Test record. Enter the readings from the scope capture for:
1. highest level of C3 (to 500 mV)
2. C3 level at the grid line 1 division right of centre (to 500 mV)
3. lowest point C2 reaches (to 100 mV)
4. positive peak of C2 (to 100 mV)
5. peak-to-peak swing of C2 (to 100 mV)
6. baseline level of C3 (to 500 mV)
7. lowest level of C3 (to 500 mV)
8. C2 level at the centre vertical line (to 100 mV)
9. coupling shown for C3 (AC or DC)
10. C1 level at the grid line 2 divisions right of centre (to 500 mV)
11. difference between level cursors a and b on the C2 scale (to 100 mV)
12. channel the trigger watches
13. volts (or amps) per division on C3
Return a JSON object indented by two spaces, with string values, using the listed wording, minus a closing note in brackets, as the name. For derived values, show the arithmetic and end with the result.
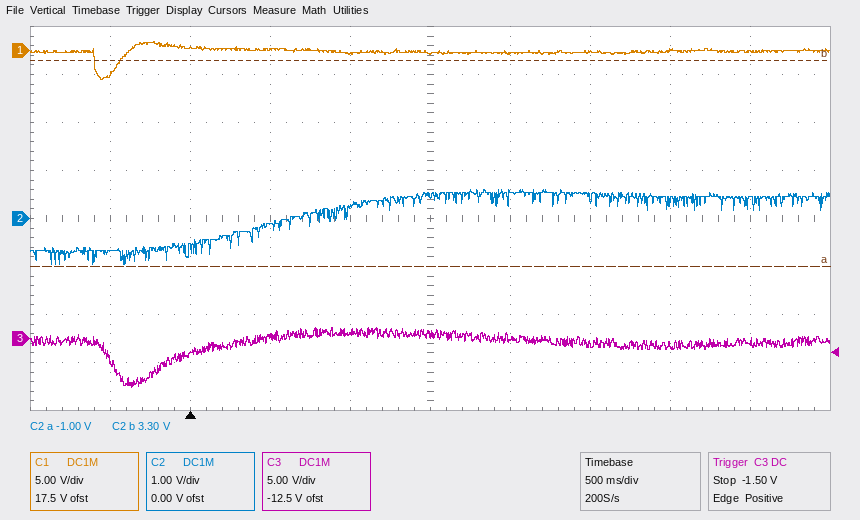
{
  "highest level of C3": "1.0 V",
  "C3 level at the grid line 1 division right of centre": "0.0 V",
  "lowest point C2 reaches": "-1.0 V",
  "positive peak of C2": "600 mV",
  "peak-to-peak swing of C2": "600 mV − (-1.0 V) = 1.6 V",
  "baseline level of C3": "-500 mV",
  "lowest level of C3": "-5.0 V",
  "C2 level at the centre vertical line": "500 mV",
  "coupling shown for C3": "DC",
  "C1 level at the grid line 2 divisions right of centre": "0.0 V",
  "difference between level cursors a and b on the C2 scale": "4.3 V",
  "channel the trigger watches": "C3",
  "volts (or amps) per division on C3": "5 V"
}
